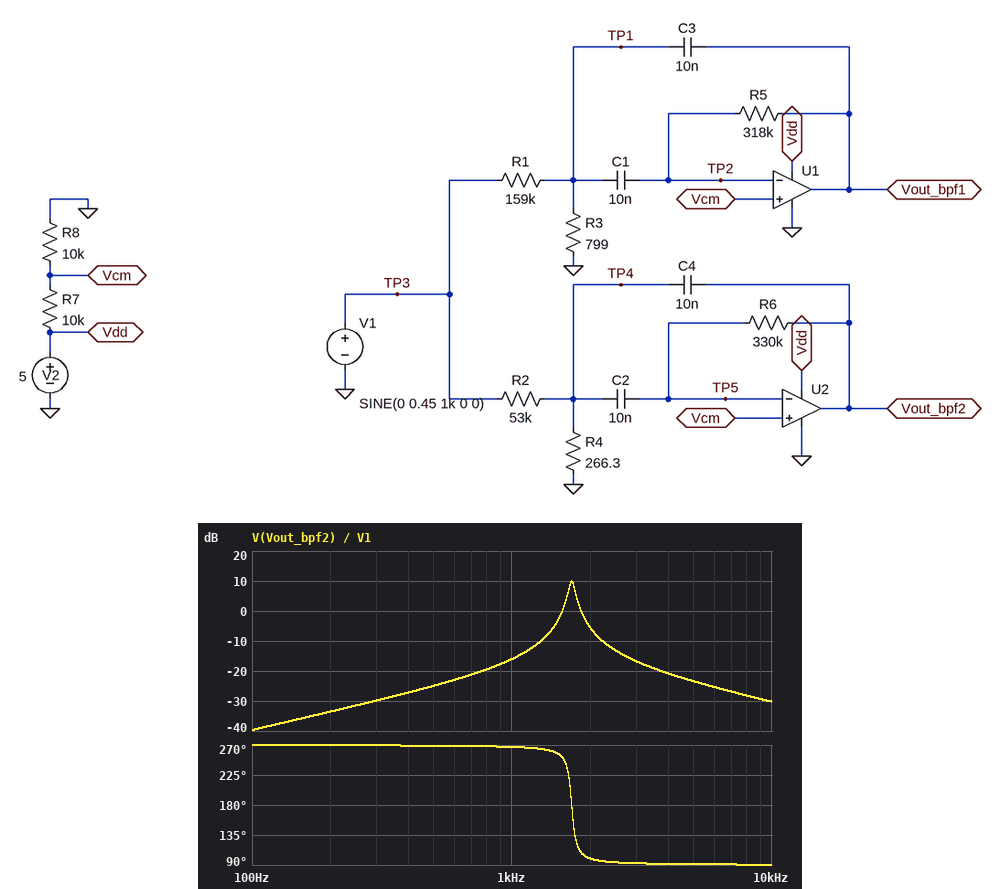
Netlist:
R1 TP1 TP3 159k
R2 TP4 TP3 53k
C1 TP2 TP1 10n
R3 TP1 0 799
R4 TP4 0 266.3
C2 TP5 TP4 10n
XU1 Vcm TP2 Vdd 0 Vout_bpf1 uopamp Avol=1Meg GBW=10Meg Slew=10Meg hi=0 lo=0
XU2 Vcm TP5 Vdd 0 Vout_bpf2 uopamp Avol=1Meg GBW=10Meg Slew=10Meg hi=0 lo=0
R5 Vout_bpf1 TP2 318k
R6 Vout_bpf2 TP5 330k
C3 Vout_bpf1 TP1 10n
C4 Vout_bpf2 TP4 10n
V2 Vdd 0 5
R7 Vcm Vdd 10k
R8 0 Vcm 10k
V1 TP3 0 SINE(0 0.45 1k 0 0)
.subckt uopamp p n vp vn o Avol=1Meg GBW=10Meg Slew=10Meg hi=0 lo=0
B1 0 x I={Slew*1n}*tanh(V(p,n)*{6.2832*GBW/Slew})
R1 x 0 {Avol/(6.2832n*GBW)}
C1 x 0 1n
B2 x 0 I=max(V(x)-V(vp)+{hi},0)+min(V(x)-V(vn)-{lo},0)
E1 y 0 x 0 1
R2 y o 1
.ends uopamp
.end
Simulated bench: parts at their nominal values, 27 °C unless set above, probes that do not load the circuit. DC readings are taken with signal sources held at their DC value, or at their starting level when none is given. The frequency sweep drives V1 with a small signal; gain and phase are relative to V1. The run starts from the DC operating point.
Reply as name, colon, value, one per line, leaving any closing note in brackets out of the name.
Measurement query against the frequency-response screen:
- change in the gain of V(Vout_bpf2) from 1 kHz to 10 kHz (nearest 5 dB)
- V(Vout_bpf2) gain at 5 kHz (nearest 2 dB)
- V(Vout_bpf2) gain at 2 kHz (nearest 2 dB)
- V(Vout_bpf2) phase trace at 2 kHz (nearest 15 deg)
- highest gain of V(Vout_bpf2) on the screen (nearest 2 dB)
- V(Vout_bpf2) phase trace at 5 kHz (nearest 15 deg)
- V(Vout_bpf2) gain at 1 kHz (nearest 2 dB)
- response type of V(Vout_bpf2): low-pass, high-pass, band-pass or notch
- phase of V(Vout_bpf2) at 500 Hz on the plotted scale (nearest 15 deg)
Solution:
change in the gain of V(Vout_bpf2) from 1 kHz to 10 kHz: -15 dB
V(Vout_bpf2) gain at 5 kHz: -24 dB
V(Vout_bpf2) gain at 2 kHz: -6 dB
V(Vout_bpf2) phase trace at 2 kHz: 105 deg
highest gain of V(Vout_bpf2) on the screen: 10 dB
V(Vout_bpf2) phase trace at 5 kHz: 90 deg
V(Vout_bpf2) gain at 1 kHz: -16 dB
response type of V(Vout_bpf2): low-pass, high-pass, band-pass or notch: band-pass
phase of V(Vout_bpf2) at 500 Hz on the plotted scale: 270 deg
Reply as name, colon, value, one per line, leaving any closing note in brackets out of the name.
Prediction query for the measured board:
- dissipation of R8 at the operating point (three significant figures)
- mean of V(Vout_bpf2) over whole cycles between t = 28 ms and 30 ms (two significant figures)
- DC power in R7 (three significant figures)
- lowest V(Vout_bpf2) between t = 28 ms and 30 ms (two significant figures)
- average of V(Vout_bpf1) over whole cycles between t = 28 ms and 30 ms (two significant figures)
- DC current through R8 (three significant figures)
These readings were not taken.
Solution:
dissipation of R8 at the operating point: 625 µW
mean of V(Vout_bpf2) over whole cycles between t = 28 ms and 30 ms: 2.5 V
DC power in R7: 625 µW
lowest V(Vout_bpf2) between t = 28 ms and 30 ms: 2.4 V
average of V(Vout_bpf1) over whole cycles between t = 28 ms and 30 ms: 2.5 V
DC current through R8: 250 µA
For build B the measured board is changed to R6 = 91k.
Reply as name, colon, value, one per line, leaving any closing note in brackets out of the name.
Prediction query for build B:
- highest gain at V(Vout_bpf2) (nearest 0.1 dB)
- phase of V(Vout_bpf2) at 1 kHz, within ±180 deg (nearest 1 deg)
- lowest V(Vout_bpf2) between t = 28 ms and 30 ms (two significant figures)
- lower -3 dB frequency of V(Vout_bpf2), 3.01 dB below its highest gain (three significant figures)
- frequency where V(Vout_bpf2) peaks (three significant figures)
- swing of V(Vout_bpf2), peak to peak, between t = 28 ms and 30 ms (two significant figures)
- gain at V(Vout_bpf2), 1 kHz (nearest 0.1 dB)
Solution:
highest gain at V(Vout_bpf2): -1.3 dB
phase of V(Vout_bpf2) at 1 kHz, within ±180 deg: -92 deg
lowest V(Vout_bpf2) between t = 28 ms and 30 ms: 2.5 V
lower -3 dB frequency of V(Vout_bpf2), 3.01 dB below its highest gain: 3.06 kHz
frequency where V(Vout_bpf2) peaks: 3.23 kHz
swing of V(Vout_bpf2), peak to peak, between t = 28 ms and 30 ms: 28 mV
gain at V(Vout_bpf2), 1 kHz: -30.0 dB
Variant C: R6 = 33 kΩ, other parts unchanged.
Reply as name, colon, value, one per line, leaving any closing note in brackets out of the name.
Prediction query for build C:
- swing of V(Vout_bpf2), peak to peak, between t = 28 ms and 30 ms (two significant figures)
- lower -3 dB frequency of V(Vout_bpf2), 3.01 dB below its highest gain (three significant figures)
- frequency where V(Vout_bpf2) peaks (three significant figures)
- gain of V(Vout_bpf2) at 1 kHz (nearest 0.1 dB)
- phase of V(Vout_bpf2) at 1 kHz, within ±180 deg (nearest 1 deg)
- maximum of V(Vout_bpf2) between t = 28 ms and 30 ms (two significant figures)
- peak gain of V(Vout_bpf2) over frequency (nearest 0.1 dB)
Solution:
swing of V(Vout_bpf2), peak to peak, between t = 28 ms and 30 ms: 9.7 mV
lower -3 dB frequency of V(Vout_bpf2), 3.01 dB below its highest gain: 4.91 kHz
frequency where V(Vout_bpf2) peaks: 5.37 kHz
gain of V(Vout_bpf2) at 1 kHz: -39.4 dB
phase of V(Vout_bpf2) at 1 kHz, within ±180 deg: -92 deg
maximum of V(Vout_bpf2) between t = 28 ms and 30 ms: 2.5 V
peak gain of V(Vout_bpf2) over frequency: -10.1 dB
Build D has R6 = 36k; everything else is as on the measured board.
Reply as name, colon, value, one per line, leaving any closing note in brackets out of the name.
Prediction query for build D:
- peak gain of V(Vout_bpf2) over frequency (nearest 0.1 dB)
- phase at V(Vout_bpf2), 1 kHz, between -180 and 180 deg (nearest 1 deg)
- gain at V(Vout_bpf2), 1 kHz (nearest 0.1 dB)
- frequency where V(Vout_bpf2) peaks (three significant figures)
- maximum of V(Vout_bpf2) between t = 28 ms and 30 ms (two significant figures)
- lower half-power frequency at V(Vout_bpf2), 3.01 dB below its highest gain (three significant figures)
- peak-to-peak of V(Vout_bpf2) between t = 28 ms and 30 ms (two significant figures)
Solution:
peak gain of V(Vout_bpf2) over frequency: -9.4 dB
phase at V(Vout_bpf2), 1 kHz, between -180 and 180 deg: -92 deg
gain at V(Vout_bpf2), 1 kHz: -38.6 dB
frequency where V(Vout_bpf2) peaks: 5.14 kHz
maximum of V(Vout_bpf2) between t = 28 ms and 30 ms: 2.5 V
lower half-power frequency at V(Vout_bpf2), 3.01 dB below its highest gain: 4.72 kHz
peak-to-peak of V(Vout_bpf2) between t = 28 ms and 30 ms: 11 mV
